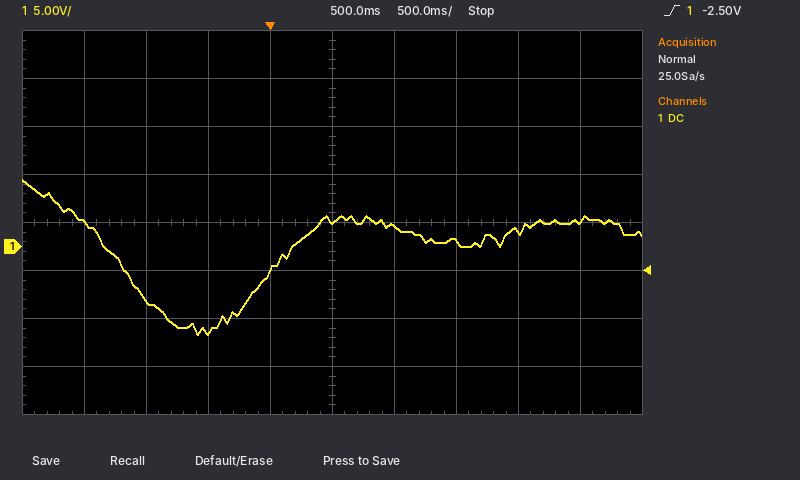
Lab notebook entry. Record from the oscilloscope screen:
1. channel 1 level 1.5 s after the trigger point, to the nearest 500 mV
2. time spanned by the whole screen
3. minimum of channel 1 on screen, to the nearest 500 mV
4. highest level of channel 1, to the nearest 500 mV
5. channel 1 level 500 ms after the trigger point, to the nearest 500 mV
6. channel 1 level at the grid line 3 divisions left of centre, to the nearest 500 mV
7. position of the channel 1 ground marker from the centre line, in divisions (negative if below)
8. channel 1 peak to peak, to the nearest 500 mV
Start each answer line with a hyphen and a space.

- 500 mV
- 5 s
- -9.0 V
- 7.0 V
- 2.5 V
- -5.5 V
- -0.5 div
- 16.0 V
